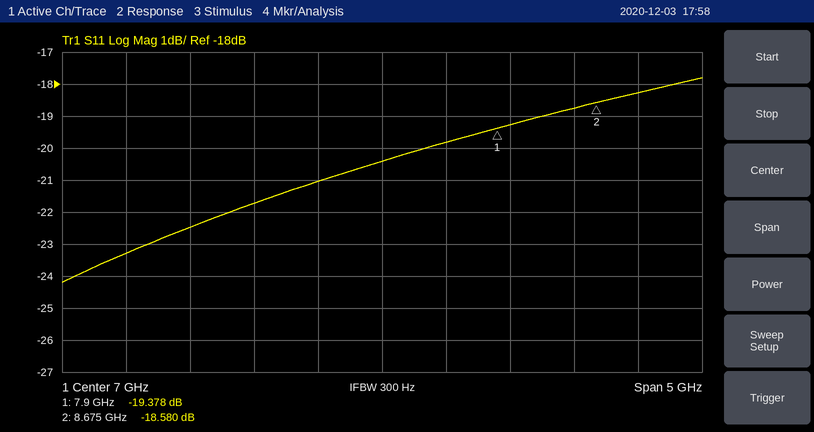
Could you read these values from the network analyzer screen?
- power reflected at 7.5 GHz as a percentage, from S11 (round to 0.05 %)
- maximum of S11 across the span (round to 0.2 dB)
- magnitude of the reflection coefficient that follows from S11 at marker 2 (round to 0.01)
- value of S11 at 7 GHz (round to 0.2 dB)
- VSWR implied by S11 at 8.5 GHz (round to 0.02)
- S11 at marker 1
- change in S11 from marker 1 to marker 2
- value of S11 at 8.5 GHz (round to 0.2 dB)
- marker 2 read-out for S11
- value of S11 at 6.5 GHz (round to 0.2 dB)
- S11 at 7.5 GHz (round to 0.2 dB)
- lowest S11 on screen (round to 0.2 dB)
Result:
1.05 %
-17.8 dB
0.12
-20.4 dB
1.26
-19.378 dB
0.798 dB
-18.8 dB
-18.580 dB
-21.0 dB
-19.8 dB
-24.2 dB
